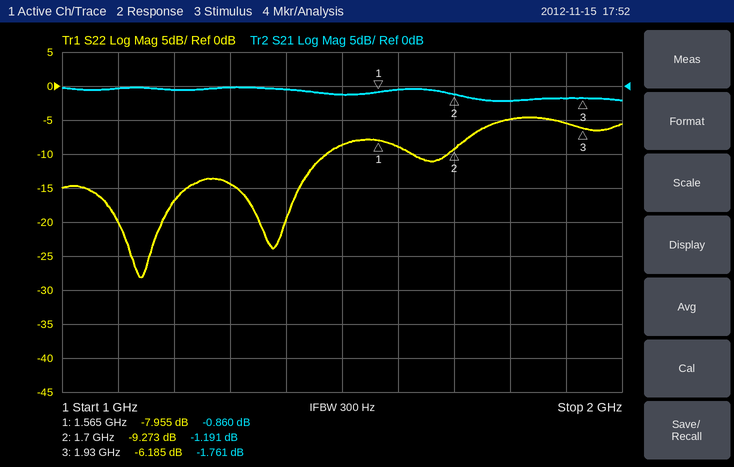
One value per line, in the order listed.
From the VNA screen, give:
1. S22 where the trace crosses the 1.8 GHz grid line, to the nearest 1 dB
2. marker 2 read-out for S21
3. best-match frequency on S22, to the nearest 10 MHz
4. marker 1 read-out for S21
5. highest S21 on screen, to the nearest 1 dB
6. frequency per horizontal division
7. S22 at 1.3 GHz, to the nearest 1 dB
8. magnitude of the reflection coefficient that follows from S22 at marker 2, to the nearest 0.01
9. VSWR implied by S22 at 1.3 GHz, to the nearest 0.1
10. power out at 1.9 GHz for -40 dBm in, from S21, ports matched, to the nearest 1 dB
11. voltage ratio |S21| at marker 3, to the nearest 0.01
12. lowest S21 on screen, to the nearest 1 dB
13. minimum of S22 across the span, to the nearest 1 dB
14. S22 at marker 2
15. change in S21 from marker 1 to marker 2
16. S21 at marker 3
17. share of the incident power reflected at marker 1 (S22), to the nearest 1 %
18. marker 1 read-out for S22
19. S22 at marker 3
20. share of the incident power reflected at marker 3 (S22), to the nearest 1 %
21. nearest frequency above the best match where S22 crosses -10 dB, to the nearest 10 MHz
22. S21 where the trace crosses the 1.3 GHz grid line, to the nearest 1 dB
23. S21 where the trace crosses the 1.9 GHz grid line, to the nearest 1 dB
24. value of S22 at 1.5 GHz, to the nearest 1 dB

-5 dB
-1.191 dB
1.14 GHz
-0.860 dB
0 dB
100 MHz
-14 dB
0.34
1.5
-42 dBm
0.82
-2 dB
-28 dB
-9.273 dB
-0.331 dB
-1.761 dB
16 %
-7.955 dB
-6.185 dB
24 %
1.47 GHz
0 dB
-2 dB
-9 dB
